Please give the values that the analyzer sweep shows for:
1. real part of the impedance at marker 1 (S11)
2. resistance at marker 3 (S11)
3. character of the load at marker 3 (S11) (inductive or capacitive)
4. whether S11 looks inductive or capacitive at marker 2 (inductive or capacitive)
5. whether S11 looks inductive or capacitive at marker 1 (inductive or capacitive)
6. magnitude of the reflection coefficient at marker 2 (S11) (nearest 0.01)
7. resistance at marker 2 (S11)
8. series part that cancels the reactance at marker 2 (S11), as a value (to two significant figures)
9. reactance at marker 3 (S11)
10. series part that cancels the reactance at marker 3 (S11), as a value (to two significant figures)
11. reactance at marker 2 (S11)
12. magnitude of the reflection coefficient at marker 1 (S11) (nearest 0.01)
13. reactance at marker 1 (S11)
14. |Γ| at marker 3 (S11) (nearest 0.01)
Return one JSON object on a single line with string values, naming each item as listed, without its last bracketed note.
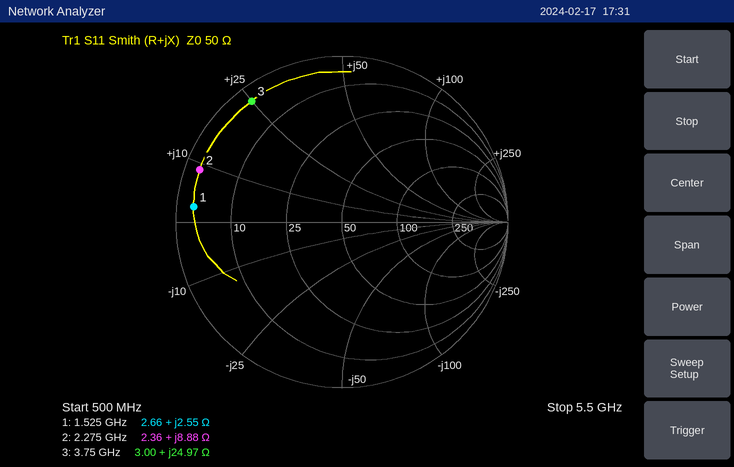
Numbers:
{"real part of the impedance at marker 1": "2.66 Ω", "resistance at marker 3": "3.00 Ω", "character of the load at marker 3 (S11)": "inductive", "whether S11 looks inductive or capacitive at marker 2": "inductive", "whether S11 looks inductive or capacitive at marker 1": "inductive", "magnitude of the reflection coefficient at marker 2 (S11)": "0.91", "resistance at marker 2": "2.36 Ω", "series part that cancels the reactance at marker 2 (S11), as a value": "7.9 pF", "reactance at marker 3": "+24.97 Ω", "series part that cancels the reactance at marker 3 (S11), as a value": "1.7 pF", "reactance at marker 2": "+8.88 Ω", "magnitude of the reflection coefficient at marker 1 (S11)": "0.90", "reactance at marker 1": "+2.55 Ω", "|Γ| at marker 3 (S11)": "0.91"}
